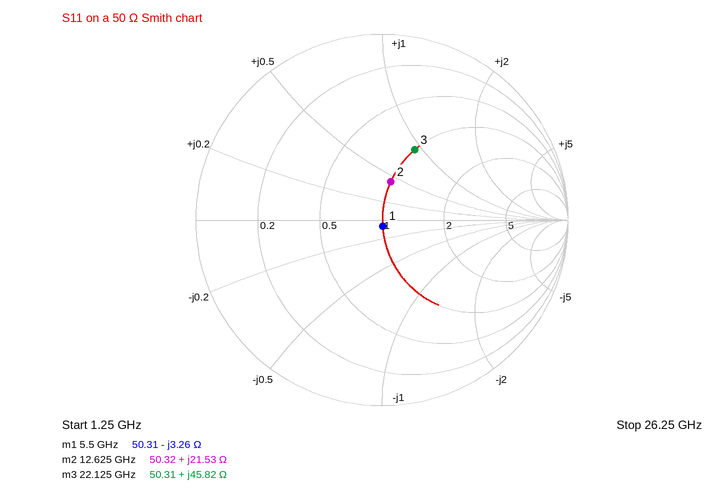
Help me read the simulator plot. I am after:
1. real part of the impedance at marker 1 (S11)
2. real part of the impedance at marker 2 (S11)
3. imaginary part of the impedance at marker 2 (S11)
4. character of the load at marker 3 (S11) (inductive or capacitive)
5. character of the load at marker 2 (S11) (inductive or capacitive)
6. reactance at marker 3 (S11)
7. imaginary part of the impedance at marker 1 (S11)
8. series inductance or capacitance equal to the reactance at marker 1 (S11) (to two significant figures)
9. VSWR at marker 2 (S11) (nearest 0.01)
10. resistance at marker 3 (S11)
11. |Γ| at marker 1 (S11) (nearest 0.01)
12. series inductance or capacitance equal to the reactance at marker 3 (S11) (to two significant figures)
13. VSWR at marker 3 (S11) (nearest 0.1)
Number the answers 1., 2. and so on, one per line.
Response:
1. 50.31 Ω
2. 50.32 Ω
3. +21.53 Ω
4. inductive
5. inductive
6. +45.82 Ω
7. -3.26 Ω
8. 8.9 pF
9. 1.53
10. 50.31 Ω
11. 0.03
12. 330 pH
13. 2.4
